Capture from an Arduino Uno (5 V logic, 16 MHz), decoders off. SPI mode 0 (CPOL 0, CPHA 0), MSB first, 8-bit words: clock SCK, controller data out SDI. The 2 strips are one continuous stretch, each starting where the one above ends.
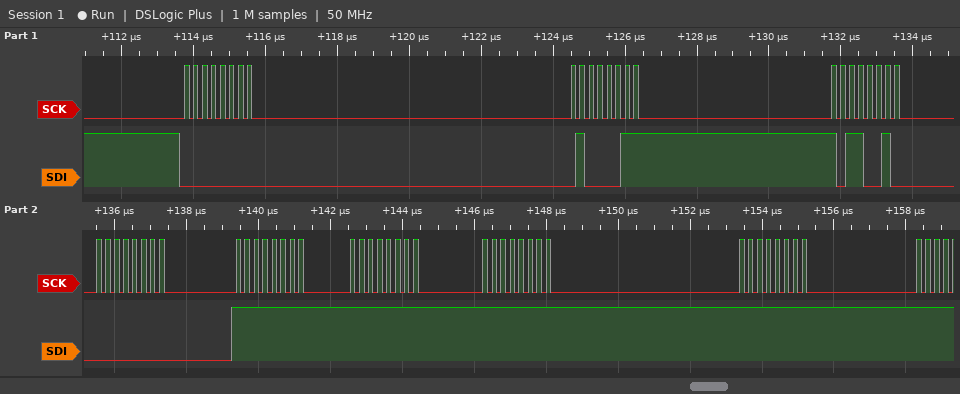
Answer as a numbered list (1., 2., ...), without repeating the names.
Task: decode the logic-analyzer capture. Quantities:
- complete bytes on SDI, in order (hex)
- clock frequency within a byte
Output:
1. 00 43 B2 00 FF FF FF FF
2. 4 MHz
